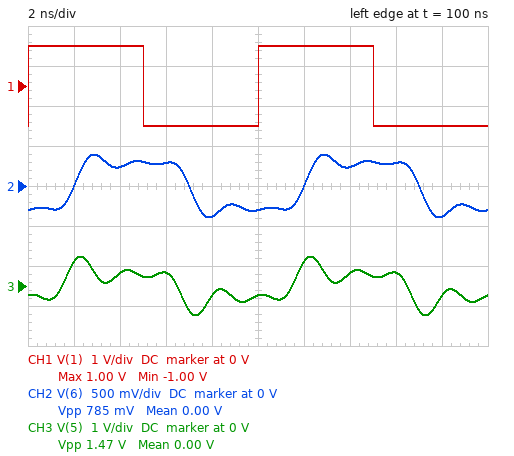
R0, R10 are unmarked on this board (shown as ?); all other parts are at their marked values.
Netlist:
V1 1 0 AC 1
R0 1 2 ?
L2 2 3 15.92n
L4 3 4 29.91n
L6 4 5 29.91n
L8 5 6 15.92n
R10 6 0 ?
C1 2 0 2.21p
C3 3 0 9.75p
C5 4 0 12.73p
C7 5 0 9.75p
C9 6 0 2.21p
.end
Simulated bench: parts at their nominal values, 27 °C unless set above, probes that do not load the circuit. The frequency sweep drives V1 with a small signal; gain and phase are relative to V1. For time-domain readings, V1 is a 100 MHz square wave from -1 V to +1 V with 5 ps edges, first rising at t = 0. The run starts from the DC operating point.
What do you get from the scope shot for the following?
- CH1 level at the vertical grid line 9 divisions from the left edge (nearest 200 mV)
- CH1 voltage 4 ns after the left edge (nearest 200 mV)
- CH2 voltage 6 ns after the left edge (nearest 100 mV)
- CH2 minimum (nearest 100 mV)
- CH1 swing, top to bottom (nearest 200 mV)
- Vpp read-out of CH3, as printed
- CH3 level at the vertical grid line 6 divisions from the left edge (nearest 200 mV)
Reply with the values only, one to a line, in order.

-1.0 V
1.0 V
300 mV
-400 mV
2.0 V
1.47 V
600 mV
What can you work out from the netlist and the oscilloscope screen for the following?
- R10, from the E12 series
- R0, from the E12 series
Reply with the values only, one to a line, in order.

18 Ω
39 Ω
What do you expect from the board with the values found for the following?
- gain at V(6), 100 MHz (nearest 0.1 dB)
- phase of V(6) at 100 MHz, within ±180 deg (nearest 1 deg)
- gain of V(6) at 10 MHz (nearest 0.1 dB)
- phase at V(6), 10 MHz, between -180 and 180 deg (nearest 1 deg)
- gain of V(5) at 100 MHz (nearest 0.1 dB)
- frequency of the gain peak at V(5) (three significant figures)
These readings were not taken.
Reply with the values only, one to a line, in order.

-10.9 dB
-69 deg
-10.0 dB
-7 deg
-9.8 dB
519 MHz
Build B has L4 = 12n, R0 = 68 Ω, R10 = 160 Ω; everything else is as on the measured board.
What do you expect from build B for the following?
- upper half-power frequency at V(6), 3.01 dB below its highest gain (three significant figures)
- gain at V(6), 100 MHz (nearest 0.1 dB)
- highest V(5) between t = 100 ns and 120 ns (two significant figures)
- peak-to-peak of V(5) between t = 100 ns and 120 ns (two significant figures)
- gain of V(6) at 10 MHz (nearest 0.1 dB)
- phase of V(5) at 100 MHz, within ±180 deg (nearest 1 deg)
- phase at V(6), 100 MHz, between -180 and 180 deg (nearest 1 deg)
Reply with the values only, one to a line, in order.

378 MHz
-4.8 dB
710 mV
1.4 V
-3.1 dB
-61 deg
-64 deg
